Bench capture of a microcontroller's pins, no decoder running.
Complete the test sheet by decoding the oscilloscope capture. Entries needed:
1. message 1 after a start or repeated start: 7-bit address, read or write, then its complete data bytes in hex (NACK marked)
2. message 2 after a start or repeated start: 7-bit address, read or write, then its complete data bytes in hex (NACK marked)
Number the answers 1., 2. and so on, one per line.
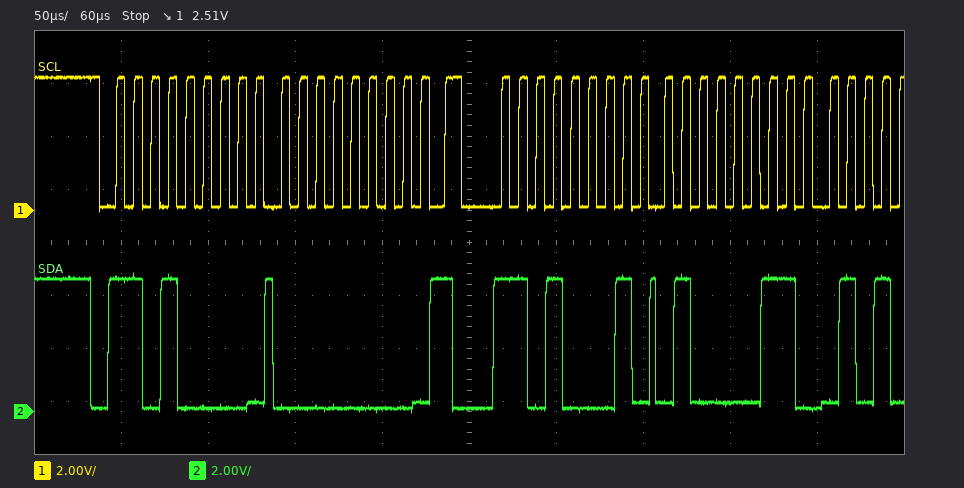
1. 0x68 write: 00
2. 0x68 read: 43
